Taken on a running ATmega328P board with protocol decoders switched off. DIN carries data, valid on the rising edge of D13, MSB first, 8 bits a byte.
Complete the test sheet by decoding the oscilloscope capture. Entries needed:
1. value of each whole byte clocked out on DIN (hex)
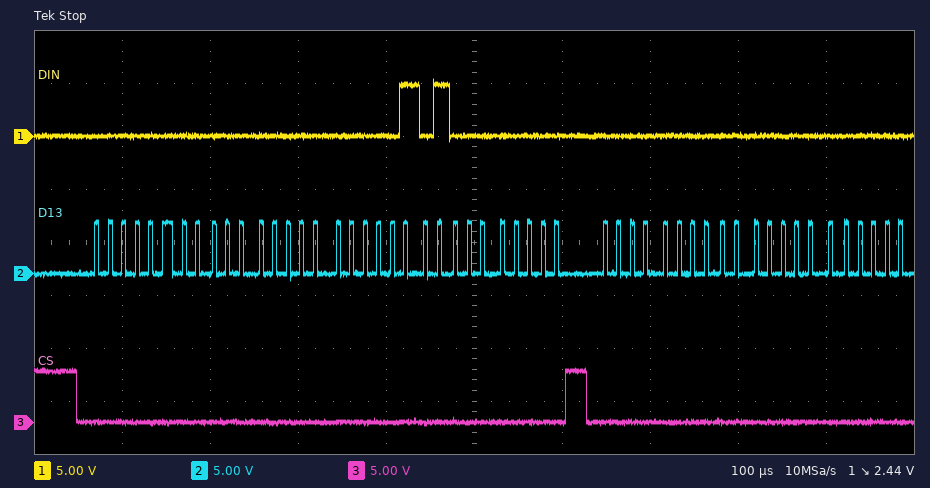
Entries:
00 00 05 00 00 00
